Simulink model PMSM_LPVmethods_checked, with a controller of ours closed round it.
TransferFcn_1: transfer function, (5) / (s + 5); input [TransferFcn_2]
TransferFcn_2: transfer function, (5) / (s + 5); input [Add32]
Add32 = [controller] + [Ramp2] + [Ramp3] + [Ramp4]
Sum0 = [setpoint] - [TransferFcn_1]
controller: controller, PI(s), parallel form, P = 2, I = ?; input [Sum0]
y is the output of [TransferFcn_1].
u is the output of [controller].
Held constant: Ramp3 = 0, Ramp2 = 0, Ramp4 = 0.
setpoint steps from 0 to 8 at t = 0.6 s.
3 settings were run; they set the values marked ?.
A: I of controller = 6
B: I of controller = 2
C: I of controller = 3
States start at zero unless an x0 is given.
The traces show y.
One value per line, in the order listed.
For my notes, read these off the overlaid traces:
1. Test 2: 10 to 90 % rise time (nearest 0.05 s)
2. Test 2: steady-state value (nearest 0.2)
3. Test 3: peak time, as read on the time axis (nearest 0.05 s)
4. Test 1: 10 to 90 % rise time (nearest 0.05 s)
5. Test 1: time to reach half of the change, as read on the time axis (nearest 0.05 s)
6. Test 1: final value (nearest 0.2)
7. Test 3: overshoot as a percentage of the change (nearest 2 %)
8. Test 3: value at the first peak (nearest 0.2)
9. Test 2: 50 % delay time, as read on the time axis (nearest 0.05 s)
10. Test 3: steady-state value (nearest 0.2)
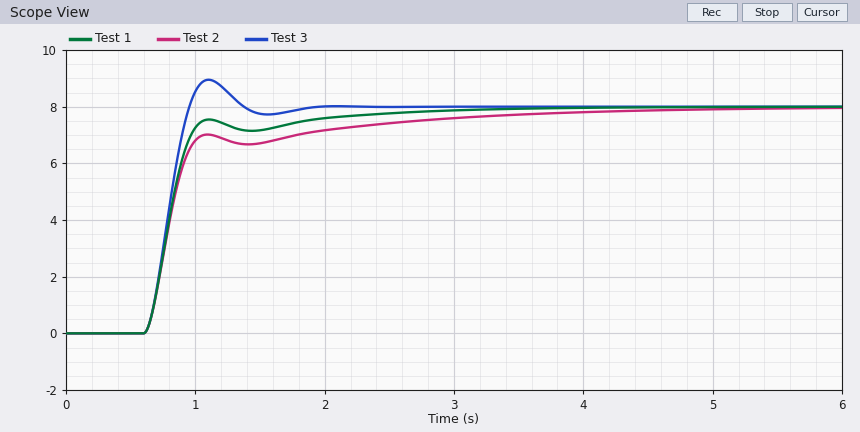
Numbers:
1.40 s
8.0
1.10 s
0.30 s
0.80 s
8.0
12 %
9.0
0.80 s
8.0
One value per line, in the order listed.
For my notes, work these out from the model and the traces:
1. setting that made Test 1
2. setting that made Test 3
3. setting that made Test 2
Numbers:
C
A
B
